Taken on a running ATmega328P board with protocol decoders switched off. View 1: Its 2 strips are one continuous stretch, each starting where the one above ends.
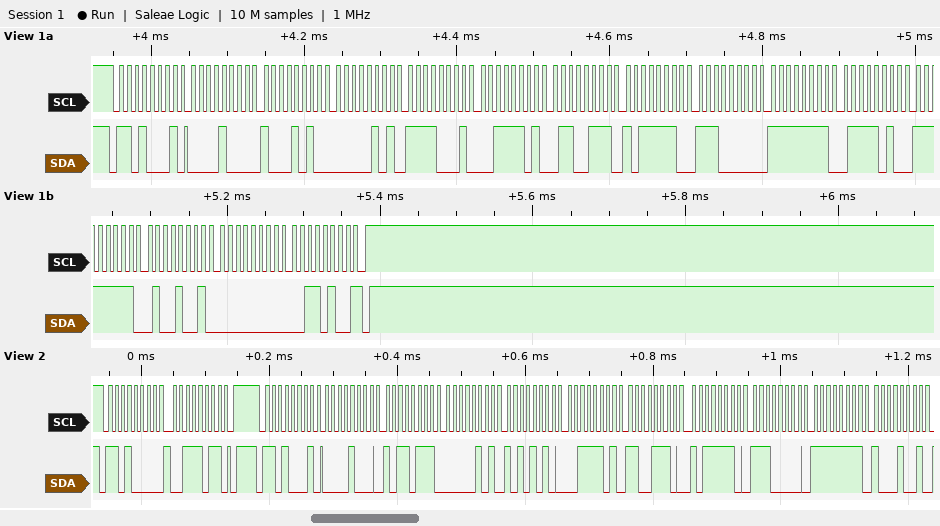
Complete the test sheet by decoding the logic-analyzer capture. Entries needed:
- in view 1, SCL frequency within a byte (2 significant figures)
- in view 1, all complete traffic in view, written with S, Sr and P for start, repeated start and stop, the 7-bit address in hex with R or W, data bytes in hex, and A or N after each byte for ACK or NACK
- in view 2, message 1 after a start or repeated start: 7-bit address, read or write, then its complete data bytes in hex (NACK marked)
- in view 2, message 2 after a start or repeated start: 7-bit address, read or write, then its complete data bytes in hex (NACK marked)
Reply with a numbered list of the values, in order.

1. 100 kHz
2. S 68R A 08 A 8A A 05 A F1 A 3D A 67 A BE A E0 A FF A 7A A FF A 49 A 00 A 34 N P
3. 0x68 write: 3B
4. 0x68 read: 08 B7 05 AA 3D CE BE E0 FF 89
